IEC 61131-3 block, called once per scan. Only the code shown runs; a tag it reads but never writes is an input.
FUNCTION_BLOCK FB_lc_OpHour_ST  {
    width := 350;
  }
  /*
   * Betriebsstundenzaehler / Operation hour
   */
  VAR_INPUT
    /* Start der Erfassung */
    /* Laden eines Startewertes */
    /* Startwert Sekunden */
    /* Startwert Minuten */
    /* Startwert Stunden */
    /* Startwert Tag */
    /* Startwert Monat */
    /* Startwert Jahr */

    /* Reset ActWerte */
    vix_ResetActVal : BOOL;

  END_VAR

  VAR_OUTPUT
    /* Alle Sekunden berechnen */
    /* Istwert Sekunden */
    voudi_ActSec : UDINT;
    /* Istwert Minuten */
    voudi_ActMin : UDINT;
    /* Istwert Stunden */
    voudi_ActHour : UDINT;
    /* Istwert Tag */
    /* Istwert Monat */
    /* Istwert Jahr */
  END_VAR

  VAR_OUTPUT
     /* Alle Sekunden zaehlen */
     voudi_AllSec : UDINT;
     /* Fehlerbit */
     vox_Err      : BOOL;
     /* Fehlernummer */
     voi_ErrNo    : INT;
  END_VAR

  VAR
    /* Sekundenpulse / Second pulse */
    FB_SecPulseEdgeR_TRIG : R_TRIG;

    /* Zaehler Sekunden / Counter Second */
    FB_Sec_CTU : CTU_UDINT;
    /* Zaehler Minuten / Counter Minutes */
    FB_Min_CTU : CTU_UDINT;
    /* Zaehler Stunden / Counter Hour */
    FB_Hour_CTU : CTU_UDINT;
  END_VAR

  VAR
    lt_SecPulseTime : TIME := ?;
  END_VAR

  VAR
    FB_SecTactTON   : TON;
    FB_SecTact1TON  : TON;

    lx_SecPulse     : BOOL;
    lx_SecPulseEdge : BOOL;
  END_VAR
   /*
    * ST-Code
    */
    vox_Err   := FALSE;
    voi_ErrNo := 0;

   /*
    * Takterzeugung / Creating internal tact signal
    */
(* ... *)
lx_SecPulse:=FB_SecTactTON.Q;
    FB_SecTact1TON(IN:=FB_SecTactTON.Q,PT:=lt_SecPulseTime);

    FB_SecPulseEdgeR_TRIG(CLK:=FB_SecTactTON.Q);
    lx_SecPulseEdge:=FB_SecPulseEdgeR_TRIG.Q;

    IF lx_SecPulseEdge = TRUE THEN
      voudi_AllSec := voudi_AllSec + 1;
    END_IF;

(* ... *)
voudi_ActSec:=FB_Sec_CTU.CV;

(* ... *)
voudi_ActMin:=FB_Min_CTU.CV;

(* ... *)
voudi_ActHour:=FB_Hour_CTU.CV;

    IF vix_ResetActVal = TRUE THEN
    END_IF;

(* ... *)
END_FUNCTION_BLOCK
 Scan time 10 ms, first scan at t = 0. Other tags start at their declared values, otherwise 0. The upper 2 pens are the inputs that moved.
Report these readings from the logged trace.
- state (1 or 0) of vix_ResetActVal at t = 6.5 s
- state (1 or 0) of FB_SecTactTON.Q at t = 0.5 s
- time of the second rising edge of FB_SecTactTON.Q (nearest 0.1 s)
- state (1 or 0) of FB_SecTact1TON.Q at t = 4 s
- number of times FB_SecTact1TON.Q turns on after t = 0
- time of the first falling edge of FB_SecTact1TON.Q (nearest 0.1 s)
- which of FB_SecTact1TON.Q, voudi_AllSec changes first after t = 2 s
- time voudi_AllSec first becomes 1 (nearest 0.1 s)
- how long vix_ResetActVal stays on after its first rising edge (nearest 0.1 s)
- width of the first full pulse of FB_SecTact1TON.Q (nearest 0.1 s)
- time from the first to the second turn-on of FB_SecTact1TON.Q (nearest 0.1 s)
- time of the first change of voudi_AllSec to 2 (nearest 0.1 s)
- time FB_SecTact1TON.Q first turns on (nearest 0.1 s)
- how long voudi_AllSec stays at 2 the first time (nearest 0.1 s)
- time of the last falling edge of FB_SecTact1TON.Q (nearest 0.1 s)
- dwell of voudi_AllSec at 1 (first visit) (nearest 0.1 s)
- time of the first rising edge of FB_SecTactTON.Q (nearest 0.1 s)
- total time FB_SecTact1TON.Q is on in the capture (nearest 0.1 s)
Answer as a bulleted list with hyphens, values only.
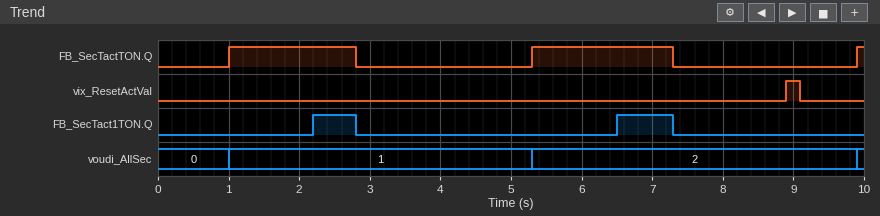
- 0
- 0
- 5.3 s
- 0
- 2
- 2.8 s
- FB_SecTact1TON.Q
- 1.0 s
- 0.2 s
- 0.6 s
- 4.3 s
- 5.3 s
- 2.2 s
- 4.6 s
- 7.3 s
- 4.3 s
- 1.0 s
- 1.4 s
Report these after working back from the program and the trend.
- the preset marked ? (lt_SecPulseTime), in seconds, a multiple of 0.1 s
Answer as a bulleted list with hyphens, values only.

- 1.2 s
